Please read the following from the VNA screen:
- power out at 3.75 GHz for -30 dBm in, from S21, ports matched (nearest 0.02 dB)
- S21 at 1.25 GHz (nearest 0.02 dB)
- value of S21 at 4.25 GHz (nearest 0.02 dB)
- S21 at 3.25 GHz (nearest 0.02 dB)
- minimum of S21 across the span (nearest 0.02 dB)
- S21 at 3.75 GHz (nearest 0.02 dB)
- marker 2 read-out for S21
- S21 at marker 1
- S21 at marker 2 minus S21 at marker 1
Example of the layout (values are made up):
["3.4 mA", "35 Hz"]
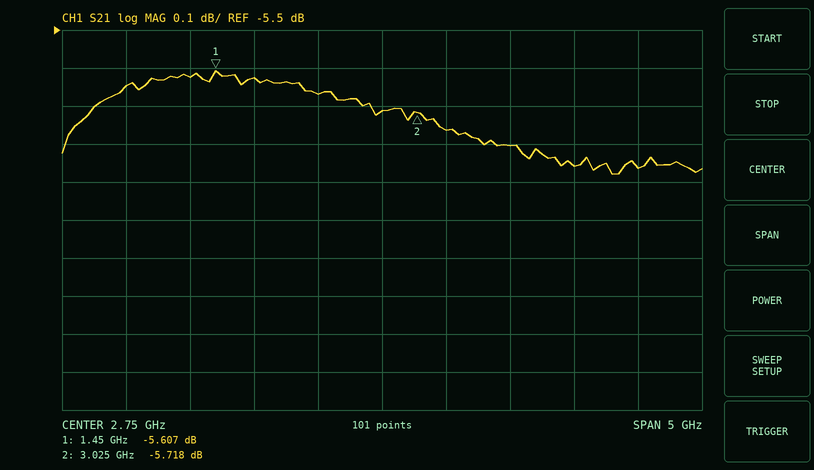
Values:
["-35.80 dBm", "-5.62 dB", "-5.86 dB", "-5.76 dB", "-5.88 dB", "-5.80 dB", "-5.718 dB", "-5.607 dB", "-0.111 dB"]
